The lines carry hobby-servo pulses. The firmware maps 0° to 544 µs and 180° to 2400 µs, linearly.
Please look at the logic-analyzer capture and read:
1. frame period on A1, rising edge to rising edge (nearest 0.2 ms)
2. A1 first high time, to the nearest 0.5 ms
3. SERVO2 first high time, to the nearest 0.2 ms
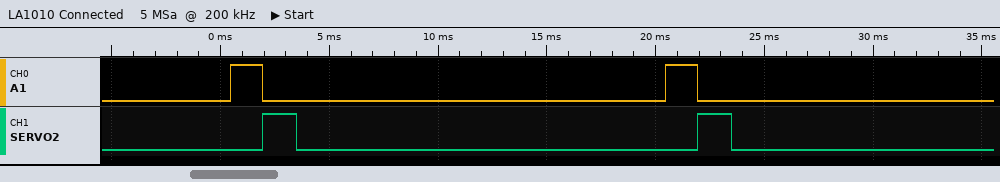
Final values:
20.0 ms
1.5 ms
1.6 ms
